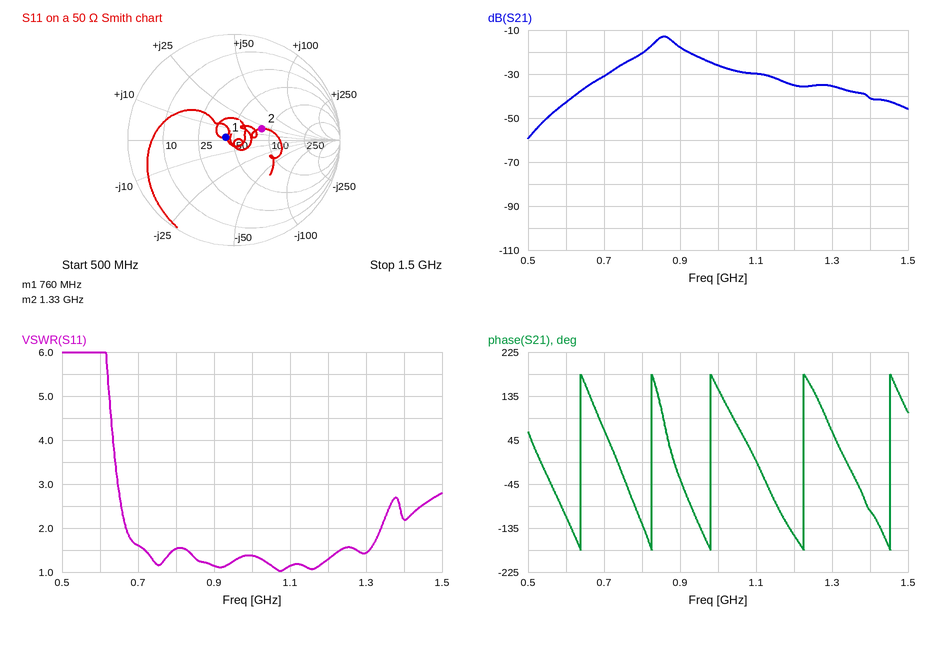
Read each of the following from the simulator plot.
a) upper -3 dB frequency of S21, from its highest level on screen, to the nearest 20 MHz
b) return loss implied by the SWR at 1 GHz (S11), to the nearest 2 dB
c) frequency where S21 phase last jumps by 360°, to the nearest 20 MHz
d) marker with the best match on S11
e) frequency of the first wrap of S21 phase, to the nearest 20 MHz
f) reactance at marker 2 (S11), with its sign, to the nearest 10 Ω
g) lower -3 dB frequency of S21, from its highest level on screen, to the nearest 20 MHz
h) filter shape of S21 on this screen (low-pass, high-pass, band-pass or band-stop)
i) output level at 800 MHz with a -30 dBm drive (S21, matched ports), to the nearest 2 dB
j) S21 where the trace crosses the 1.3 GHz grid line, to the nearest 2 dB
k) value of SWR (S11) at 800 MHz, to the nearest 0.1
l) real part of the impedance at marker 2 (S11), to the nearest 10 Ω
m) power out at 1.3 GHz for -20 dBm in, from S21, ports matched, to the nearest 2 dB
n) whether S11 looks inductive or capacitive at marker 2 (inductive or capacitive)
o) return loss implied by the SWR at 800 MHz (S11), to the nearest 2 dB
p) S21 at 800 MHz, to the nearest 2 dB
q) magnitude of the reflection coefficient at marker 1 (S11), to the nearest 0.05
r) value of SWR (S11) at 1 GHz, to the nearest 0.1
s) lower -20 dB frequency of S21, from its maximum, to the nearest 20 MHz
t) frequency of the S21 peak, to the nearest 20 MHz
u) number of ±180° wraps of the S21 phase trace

880 MHz
16 dB
1.46 GHz
marker 1
640 MHz
+20 Ω
840 MHz
band-pass
-50 dBm
-36 dB
1.5
80 Ω
-56 dBm
inductive
14 dB
-20 dB
0.10
1.4
680 MHz
860 MHz
5
